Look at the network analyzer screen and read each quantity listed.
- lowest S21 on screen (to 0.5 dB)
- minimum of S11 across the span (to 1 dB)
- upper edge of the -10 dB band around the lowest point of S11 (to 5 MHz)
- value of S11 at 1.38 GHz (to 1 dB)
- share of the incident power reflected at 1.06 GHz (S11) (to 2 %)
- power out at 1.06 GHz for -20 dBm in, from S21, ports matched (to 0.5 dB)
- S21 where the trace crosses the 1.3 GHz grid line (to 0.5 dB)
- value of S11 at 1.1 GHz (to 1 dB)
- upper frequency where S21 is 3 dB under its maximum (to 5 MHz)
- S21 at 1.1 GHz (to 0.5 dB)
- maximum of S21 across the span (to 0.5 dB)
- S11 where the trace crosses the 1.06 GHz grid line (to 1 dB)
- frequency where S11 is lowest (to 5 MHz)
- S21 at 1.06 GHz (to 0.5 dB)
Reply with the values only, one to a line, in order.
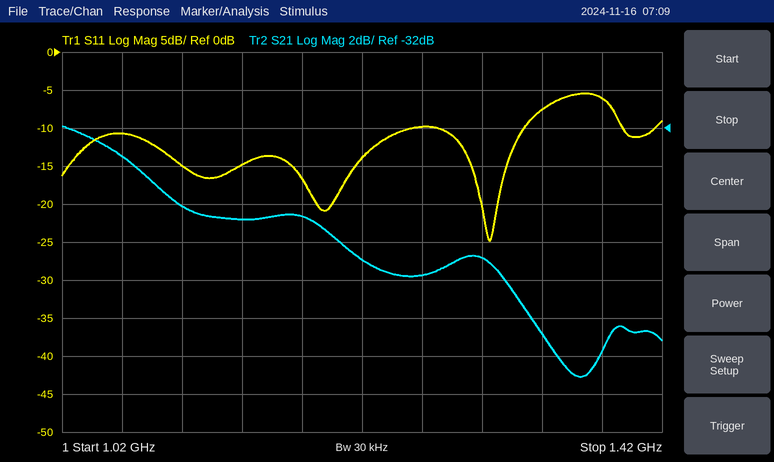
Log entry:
-45.0 dB
-25 dB
1.330 GHz
-6 dB
8 %
-53.5 dBm
-39.0 dB
-15 dB
1.080 GHz
-36.0 dB
-32.0 dB
-11 dB
1.305 GHz
-33.5 dB
